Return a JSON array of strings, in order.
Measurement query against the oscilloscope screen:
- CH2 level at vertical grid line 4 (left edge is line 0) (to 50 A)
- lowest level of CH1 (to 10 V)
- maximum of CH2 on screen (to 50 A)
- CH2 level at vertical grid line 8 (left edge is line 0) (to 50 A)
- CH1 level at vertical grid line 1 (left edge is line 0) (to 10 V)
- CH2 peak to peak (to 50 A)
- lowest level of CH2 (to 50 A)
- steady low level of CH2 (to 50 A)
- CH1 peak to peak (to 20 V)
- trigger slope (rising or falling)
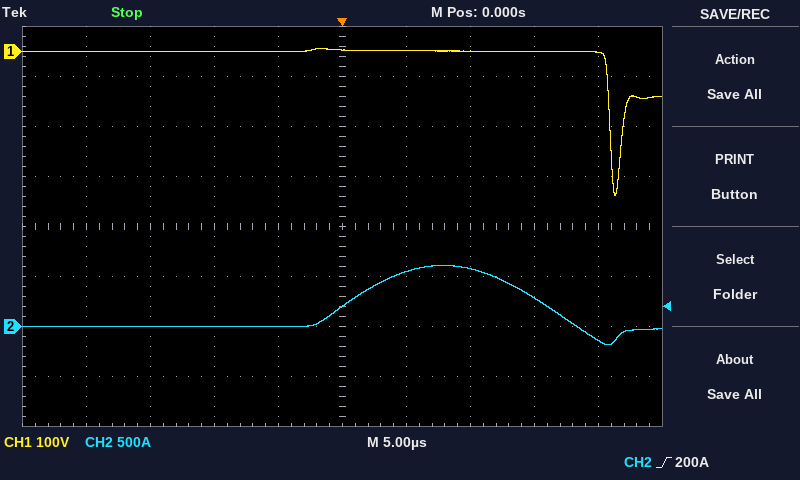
["0 A", "-290 V", "600 A", "300 A", "0 V", "800 A", "-200 A", "0 A", "300 V", "rising"]
